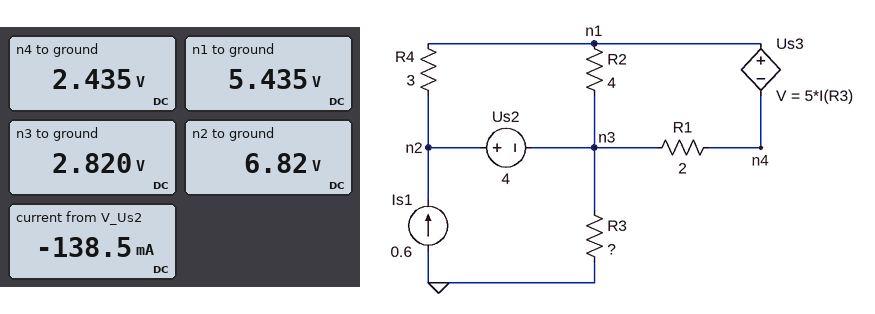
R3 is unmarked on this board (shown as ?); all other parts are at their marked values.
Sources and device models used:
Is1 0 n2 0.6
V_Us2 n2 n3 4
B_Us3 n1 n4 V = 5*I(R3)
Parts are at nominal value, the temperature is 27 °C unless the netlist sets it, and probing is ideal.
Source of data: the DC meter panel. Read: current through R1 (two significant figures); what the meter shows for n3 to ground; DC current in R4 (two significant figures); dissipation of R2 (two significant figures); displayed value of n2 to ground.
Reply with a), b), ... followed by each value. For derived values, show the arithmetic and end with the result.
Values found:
a) (2.82 V - 2.435 V) / 2 Ω = 190 mA
b) 2.820 V
c) (6.82 V - 5.435 V) / 3 Ω = 460 mA
d) (5.435 V - 2.82 V)^2 / 4 Ω = 1.7 W
e) 6.82 V
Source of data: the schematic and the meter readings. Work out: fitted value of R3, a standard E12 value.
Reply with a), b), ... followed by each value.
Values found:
a) 4.7 Ω
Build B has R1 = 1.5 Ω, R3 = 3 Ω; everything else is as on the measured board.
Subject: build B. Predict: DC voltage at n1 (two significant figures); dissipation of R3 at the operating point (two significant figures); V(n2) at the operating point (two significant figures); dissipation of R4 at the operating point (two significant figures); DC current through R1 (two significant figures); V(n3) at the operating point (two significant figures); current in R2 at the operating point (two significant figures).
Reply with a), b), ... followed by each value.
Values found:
a) 4.5 V
b) 1.1 W
c) 5.8 V
d) 590 mW
e) 220 mA
f) 1.8 V
g) 670 mA
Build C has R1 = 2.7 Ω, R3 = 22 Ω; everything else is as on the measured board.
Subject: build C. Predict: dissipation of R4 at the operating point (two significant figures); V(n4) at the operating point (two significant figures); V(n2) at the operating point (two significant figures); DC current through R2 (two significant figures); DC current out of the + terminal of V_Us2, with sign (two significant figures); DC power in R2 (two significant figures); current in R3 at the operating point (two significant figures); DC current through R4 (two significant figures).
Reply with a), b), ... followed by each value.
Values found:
a) 690 mW
b) 13 V
c) 17 V
d) 640 mA
e) -120 mA
f) 1.6 W
g) 600 mA
h) 480 mA
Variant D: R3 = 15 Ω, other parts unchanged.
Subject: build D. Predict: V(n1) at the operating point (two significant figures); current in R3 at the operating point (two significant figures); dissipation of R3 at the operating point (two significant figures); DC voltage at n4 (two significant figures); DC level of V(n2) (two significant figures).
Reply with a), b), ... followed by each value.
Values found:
a) 12 V
b) 600 mA
c) 5.4 W
d) 8.6 V
e) 13 V
